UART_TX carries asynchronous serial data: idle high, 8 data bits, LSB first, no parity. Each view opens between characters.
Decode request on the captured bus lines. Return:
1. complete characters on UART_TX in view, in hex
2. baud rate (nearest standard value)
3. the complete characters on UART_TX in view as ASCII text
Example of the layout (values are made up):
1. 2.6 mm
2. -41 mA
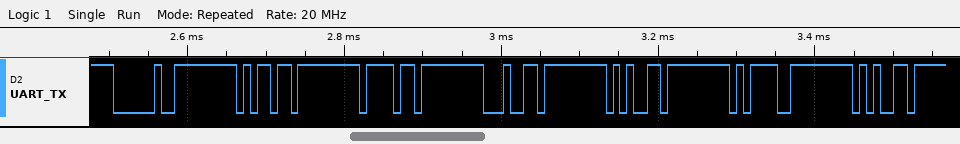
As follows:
1. 20, 6D, 6F, 64, 65, 3D, 65
2. 115200 baud
3. " mode=e"
